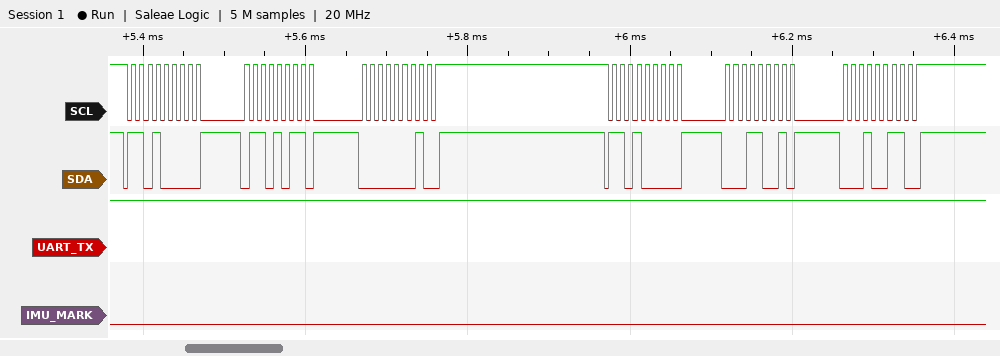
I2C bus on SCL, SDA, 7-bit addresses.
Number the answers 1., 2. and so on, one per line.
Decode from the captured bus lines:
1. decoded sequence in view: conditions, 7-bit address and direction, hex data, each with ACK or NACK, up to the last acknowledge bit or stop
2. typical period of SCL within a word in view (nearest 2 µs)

1. start, address 68 write ACK, 6B ACK, 01 ACK, stop, start, address 68 write ACK, 19 ACK, 13 ACK, stop
2. 10 µs
